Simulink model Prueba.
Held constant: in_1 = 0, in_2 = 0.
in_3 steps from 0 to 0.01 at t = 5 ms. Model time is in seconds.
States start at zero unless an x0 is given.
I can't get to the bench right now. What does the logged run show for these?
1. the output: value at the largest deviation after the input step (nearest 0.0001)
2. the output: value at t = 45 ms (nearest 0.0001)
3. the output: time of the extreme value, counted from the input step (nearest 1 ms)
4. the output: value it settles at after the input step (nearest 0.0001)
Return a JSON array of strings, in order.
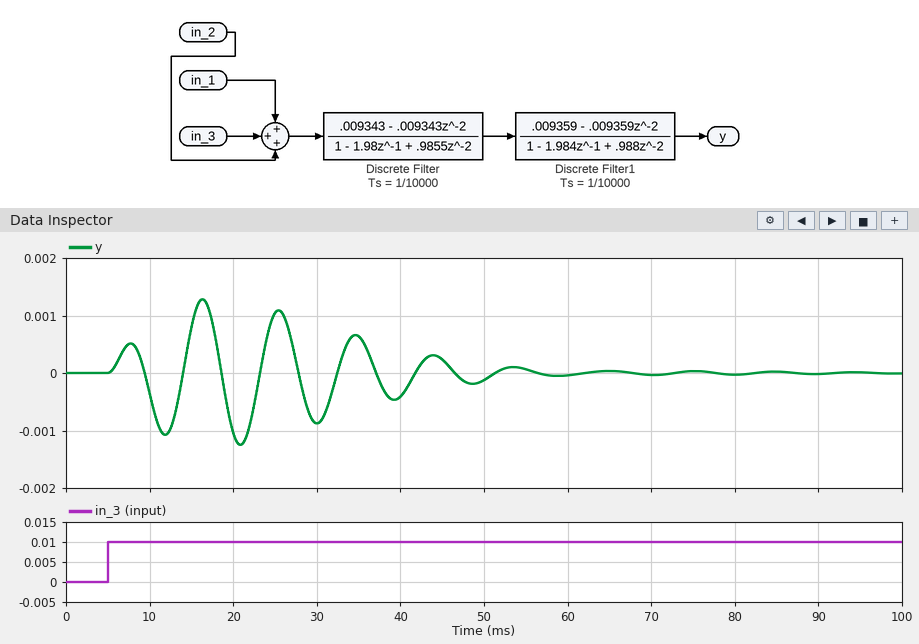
["0.0013", "0.0002", "11 ms", "0.0000"]
